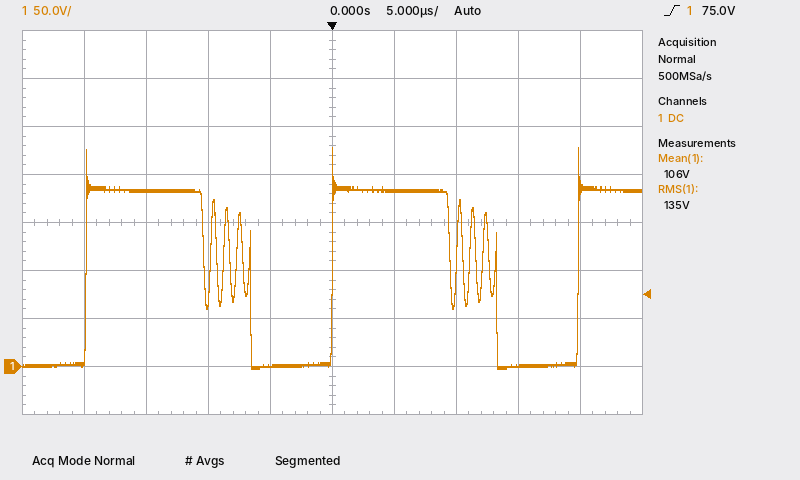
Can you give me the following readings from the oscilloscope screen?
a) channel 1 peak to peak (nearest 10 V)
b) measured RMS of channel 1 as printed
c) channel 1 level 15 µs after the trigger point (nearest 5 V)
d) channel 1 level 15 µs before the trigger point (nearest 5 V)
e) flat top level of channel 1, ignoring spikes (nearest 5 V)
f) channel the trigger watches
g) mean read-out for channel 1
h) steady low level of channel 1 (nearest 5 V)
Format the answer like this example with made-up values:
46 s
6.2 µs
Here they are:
230 V
135 V
0 V
185 V
185 V
channel 1
106 V
0 V
